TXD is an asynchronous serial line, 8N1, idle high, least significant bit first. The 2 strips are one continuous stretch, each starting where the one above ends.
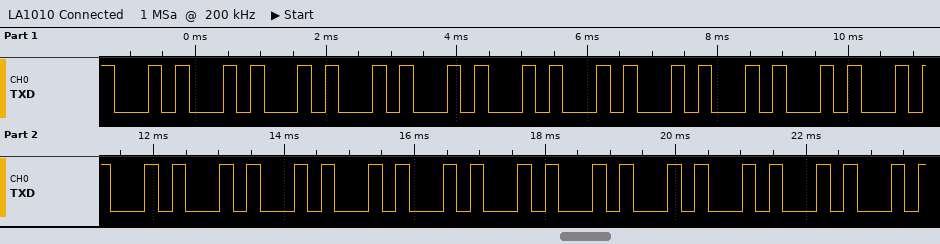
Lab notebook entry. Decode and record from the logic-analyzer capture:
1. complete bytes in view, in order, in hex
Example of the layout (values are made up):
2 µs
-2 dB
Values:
30 30 30 30 30 30 30 30 30 30 30 30 30 30 30 30 30 30 30 30 30 30
